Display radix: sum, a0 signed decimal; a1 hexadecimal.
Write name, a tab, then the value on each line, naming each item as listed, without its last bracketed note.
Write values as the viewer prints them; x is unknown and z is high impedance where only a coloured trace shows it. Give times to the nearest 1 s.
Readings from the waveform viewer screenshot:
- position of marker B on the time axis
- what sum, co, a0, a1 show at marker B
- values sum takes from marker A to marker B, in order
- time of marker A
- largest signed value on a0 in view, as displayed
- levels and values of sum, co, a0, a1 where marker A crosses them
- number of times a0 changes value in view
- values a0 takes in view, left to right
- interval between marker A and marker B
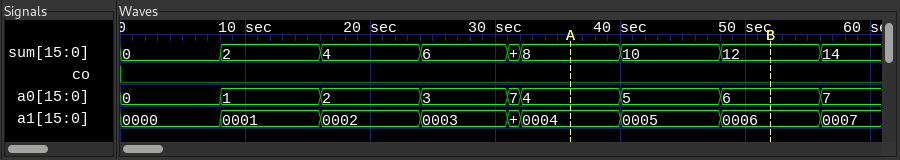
position of marker B on the time axis	52 s
what sum, co, a0, a1 show at marker B	sum=12, co=0, a0=6, a1=0006
values sum takes from marker A to marker B, in order	8, 10, 12
time of marker A	36 s
largest signed value on a0 in view, as displayed	7
levels and values of sum, co, a0, a1 where marker A crosses them	sum=8, co=0, a0=4, a1=0004
number of times a0 changes value in view	8
values a0 takes in view, left to right	0, 1, 2, 3, 7, 4, 5, 6, 7
interval between marker A and marker B	16 s
